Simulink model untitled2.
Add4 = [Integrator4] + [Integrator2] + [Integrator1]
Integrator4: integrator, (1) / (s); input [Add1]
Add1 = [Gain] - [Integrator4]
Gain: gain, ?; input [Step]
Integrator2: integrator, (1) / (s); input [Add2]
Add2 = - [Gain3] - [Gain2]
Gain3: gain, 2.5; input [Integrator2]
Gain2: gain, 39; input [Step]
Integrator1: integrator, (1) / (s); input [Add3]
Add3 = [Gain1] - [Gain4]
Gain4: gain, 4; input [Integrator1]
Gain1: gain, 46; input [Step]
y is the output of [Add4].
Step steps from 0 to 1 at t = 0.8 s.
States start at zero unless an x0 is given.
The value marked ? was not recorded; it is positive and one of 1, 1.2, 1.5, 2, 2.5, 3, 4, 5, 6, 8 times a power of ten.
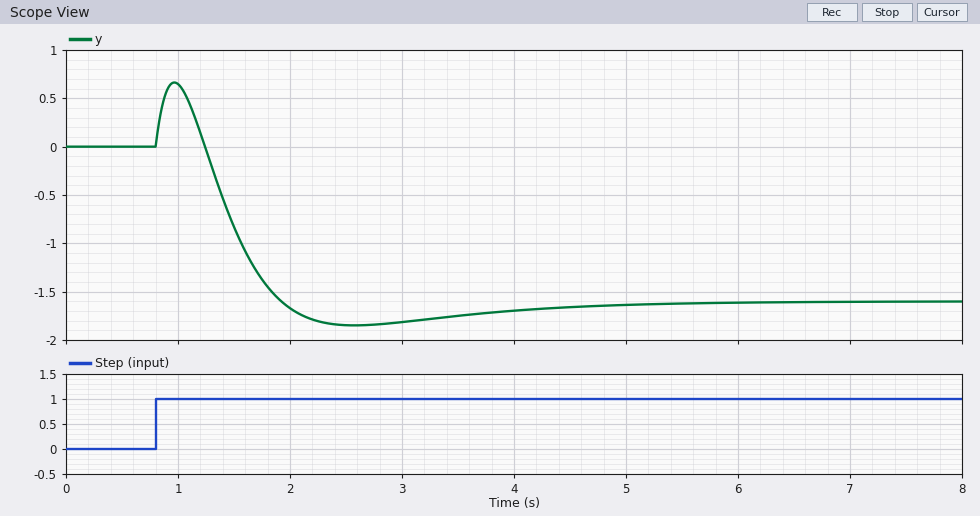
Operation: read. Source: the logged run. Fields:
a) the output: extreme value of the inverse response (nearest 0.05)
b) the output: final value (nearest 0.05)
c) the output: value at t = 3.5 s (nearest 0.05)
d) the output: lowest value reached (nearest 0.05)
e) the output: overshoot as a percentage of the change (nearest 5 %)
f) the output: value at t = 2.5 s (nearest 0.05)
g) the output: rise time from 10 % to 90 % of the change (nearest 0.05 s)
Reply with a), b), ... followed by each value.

a) 0.65
b) -1.60
c) -1.75
d) -1.85
e) 15 %
f) -1.85
g) 0.50 s
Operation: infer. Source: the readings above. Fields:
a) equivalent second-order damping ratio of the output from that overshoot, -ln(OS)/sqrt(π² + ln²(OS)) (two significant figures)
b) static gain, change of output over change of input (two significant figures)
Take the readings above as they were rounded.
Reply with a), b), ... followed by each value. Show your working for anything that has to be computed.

a) ln(0.15) = -1.897; 1.897 / sqrt(9.870 + 3.599) = 0.52
b) (-1.6 - 0) / (1 - 0) = -1.6
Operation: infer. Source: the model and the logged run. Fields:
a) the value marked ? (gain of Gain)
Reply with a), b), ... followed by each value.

a) 2.5
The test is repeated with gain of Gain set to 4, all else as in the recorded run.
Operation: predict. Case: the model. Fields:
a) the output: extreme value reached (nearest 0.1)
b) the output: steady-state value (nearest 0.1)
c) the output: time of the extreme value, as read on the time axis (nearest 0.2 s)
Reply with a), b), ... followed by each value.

a) 0.9
b) -0.1
c) 1.0 s
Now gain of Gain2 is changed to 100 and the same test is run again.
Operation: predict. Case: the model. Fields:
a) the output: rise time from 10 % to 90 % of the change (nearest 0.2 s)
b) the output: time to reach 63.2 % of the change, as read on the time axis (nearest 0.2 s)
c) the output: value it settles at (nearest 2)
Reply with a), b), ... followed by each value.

a) 0.8 s
b) 1.2 s
c) -26
